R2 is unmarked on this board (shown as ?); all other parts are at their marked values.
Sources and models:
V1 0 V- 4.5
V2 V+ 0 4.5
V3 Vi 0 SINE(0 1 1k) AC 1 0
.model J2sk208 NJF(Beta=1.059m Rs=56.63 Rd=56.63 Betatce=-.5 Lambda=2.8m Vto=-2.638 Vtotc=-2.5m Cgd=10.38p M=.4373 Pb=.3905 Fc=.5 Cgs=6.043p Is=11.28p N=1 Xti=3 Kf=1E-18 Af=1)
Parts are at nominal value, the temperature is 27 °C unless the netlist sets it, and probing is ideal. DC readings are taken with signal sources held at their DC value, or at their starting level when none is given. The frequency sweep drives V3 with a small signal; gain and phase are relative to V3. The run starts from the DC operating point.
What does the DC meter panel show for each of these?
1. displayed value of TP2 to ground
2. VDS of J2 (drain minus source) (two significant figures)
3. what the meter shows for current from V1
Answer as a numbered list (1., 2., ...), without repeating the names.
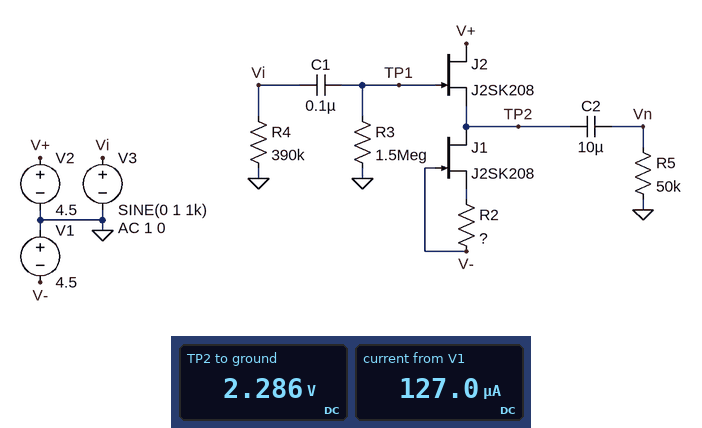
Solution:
1. 2.286 V
2. 2.2 V
3. 127.0 µA
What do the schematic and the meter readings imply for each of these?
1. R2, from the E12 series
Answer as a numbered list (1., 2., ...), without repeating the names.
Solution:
1. 18 kΩ
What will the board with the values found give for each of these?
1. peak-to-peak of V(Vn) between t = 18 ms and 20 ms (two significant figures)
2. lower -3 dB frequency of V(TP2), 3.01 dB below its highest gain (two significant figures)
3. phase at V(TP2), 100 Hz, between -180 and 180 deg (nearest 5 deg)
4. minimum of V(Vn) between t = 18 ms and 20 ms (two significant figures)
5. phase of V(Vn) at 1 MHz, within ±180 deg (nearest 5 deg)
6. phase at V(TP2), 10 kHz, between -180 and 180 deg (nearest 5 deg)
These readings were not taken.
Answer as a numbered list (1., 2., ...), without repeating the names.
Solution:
1. 1.9 V
2. 1.1 Hz
3. 0 deg
4. -970 mV
5. 0 deg
6. 0 deg
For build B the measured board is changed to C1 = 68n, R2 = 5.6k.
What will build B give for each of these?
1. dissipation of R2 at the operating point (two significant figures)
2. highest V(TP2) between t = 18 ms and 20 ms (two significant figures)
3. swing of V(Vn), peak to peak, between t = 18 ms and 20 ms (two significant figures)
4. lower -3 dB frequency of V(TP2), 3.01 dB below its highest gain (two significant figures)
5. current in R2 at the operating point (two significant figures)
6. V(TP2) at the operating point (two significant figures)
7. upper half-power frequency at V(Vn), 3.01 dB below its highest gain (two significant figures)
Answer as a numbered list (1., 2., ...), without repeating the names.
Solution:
1. 740 µW
2. 3.0 V
3. 2.0 V
4. 1.6 Hz
5. 360 µA
6. 2.0 V
7. 55 MHz
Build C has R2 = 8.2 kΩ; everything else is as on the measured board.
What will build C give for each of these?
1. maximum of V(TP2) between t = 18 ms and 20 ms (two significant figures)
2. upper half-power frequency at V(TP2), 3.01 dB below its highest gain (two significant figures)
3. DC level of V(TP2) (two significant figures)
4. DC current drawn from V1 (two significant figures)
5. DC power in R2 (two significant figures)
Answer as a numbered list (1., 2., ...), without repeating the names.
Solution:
1. 3.1 V
2. 47 MHz
3. 2.1 V
4. 260 µA
5. 550 µW
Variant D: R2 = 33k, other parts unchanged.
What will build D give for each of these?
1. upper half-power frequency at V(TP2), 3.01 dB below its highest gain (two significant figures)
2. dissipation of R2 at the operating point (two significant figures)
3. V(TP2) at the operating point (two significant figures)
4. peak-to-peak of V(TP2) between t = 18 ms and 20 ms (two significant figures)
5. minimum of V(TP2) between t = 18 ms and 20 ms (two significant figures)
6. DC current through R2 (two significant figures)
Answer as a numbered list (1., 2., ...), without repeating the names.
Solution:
1. 27 MHz
2. 170 µW
3. 2.4 V
4. 1.9 V
5. 1.4 V
6. 72 µA
